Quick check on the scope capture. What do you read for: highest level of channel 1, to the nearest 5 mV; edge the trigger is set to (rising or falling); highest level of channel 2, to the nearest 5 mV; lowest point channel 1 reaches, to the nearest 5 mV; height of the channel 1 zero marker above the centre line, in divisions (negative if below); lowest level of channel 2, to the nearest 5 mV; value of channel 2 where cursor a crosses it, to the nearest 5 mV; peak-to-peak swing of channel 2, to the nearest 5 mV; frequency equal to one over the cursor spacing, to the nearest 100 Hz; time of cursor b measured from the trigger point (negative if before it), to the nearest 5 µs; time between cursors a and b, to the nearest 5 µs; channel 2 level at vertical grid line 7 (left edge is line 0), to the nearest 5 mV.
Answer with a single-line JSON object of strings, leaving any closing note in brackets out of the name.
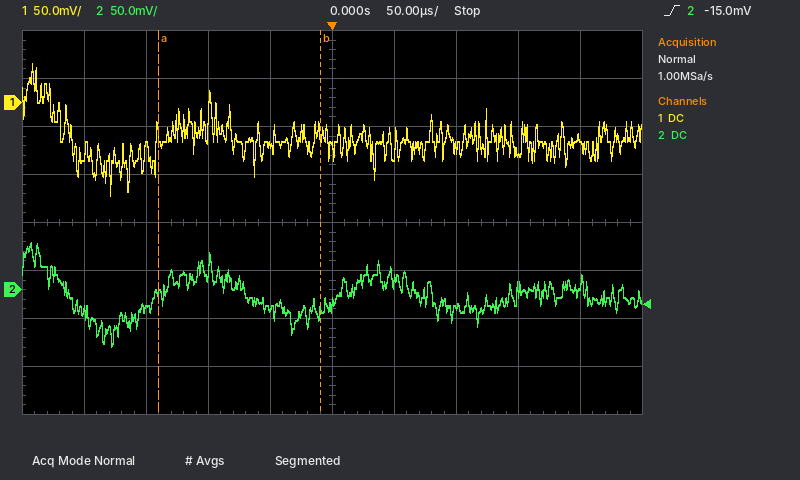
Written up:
{"highest level of channel 1, to the nearest 5 mV": "40 mV", "edge the trigger is set to": "rising", "highest level of channel 2, to the nearest 5 mV": "50 mV", "lowest point channel 1 reaches, to the nearest 5 mV": "-95 mV", "height of the channel 1 zero marker above the centre line, in divisions": "+2.5 div", "lowest level of channel 2, to the nearest 5 mV": "-60 mV", "value of channel 2 where cursor a crosses it, to the nearest 5 mV": "-5 mV", "peak-to-peak swing of channel 2, to the nearest 5 mV": "110 mV", "frequency equal to one over the cursor spacing, to the nearest 100 Hz": "7.7 kHz", "time of cursor b measured from the trigger point (negative if before it), to the nearest 5 µs": "-10 µs", "time between cursors a and b, to the nearest 5 µs": "130 µs", "channel 2 level at vertical grid line 7 (left edge is line 0), to the nearest 5 mV": "-20 mV"}
